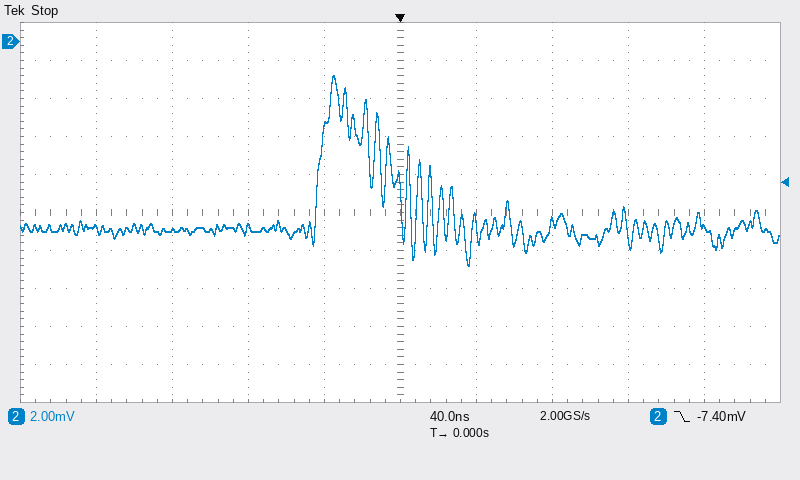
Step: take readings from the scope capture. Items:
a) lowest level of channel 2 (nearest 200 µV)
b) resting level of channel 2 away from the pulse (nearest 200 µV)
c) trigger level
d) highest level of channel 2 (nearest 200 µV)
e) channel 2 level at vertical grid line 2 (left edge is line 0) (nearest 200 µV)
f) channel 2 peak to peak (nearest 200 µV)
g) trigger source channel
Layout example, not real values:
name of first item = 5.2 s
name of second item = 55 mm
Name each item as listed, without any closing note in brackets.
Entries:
lowest level of channel 2 = -11.8 mV
resting level of channel 2 away from the pulse = -9.8 mV
trigger level = -7.40 mV
highest level of channel 2 = -1.8 mV
channel 2 level at vertical grid line 2 (left edge is line 0) = -10.0 mV
channel 2 peak to peak = 10.0 mV
trigger source channel = channel 2
